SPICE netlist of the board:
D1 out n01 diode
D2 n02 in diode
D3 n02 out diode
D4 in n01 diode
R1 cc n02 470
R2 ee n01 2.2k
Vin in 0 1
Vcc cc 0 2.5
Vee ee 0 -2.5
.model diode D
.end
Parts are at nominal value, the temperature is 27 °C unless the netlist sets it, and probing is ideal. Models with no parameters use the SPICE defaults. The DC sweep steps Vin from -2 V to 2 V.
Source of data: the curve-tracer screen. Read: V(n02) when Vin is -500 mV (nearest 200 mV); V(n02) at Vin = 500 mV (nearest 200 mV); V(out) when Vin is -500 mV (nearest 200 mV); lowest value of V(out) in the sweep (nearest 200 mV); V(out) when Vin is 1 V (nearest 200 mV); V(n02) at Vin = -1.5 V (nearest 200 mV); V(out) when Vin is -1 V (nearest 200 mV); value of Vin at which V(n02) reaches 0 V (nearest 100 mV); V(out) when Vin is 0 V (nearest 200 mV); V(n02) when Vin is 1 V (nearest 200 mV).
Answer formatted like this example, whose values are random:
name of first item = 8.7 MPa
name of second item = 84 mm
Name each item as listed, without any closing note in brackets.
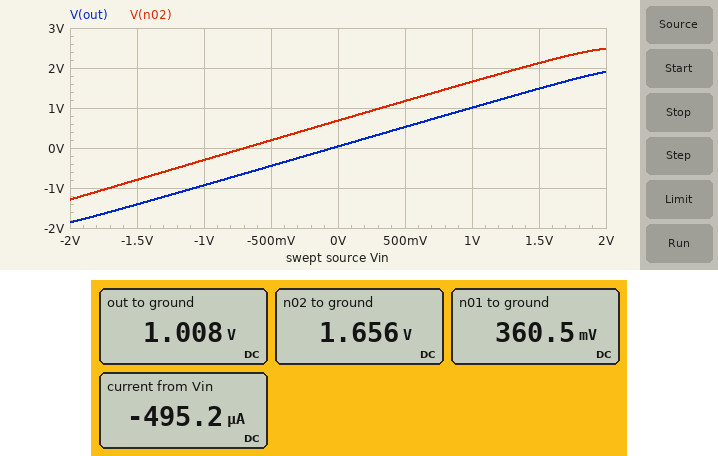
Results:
V(n02) when Vin is -500 mV = 200 mV
V(n02) at Vin = 500 mV = 1.2 V
V(out) when Vin is -500 mV = -400 mV
lowest value of V(out) in the sweep = -1.8 V
V(out) when Vin is 1 V = 1.0 V
V(n02) at Vin = -1.5 V = -800 mV
V(out) when Vin is -1 V = -1.0 V
value of Vin at which V(n02) reaches 0 V = -700 mV
V(out) when Vin is 0 V = 0 V
V(n02) when Vin is 1 V = 1.6 V
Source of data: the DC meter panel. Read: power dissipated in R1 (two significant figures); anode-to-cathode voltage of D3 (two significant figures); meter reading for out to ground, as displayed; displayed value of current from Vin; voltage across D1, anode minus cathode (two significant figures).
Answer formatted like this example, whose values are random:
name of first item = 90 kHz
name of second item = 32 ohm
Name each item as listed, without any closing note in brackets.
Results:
power dissipated in R1 = 1.5 mW
anode-to-cathode voltage of D3 = 650 mV
meter reading for out to ground, as displayed = 1.008 V
displayed value of current from Vin = -495.2 µA
voltage across D1, anode minus cathode = 650 mV
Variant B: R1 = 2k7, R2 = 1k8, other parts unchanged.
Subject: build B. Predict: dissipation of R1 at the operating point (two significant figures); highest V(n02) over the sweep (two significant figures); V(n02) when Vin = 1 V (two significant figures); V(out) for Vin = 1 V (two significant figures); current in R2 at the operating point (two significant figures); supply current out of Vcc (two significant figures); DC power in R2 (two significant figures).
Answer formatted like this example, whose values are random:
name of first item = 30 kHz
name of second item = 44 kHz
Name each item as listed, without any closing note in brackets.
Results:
dissipation of R1 at the operating point = 310 µW
highest V(n02) over the sweep = 2.4 V
V(n02) when Vin = 1 V = 1.6 V
V(out) for Vin = 1 V = 960 mV
current in R2 at the operating point = 1.6 mA
supply current out of Vcc = 340 µA
DC power in R2 = 4.5 mW
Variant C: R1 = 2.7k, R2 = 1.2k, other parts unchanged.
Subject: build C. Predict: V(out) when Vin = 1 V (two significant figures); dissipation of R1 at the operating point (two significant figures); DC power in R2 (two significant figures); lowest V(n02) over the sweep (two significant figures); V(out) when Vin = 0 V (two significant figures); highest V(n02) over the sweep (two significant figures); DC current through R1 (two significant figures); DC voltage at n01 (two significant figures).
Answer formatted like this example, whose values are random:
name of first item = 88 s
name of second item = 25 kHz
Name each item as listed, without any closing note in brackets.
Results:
V(out) when Vin = 1 V = 950 mV
dissipation of R1 at the operating point = 320 µW
DC power in R2 = 6.7 mW
lowest V(n02) over the sweep = -1.3 V
V(out) when Vin = 0 V = -20 mV
highest V(n02) over the sweep = 2.4 V
DC current through R1 = 340 µA
DC voltage at n01 = 330 mV
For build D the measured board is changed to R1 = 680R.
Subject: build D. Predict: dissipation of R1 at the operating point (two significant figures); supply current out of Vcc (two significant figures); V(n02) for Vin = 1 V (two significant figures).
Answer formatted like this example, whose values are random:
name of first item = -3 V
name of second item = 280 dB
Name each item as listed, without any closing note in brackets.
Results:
dissipation of R1 at the operating point = 1.1 mW
supply current out of Vcc = 1.3 mA
V(n02) for Vin = 1 V = 1.6 V
